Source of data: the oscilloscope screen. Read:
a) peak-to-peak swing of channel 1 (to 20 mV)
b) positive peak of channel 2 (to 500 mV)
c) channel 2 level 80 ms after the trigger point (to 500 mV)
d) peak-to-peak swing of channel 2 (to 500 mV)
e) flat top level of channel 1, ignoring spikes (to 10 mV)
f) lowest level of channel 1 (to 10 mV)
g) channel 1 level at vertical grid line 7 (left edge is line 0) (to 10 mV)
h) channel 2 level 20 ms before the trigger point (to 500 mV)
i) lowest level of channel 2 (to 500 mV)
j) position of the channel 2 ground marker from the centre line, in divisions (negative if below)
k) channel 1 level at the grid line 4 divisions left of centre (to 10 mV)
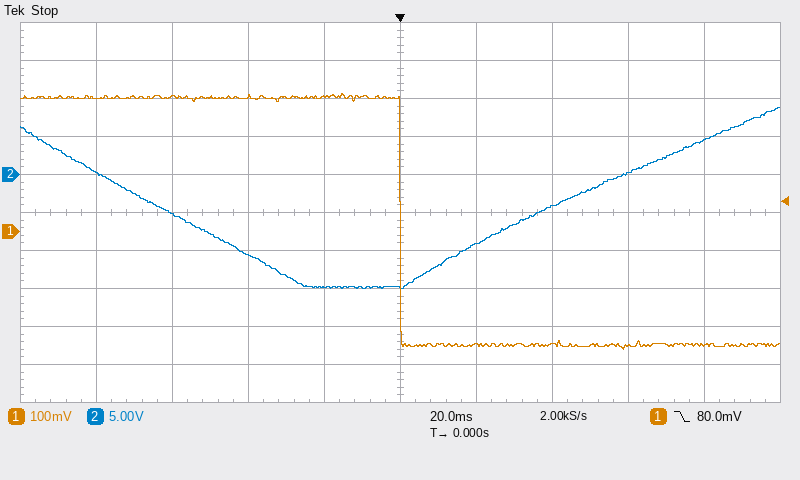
680 mV
9.0 V
4.5 V
24.0 V
350 mV
-310 mV
-300 mV
-15.0 V
-15.0 V
+1.0 div
350 mV
